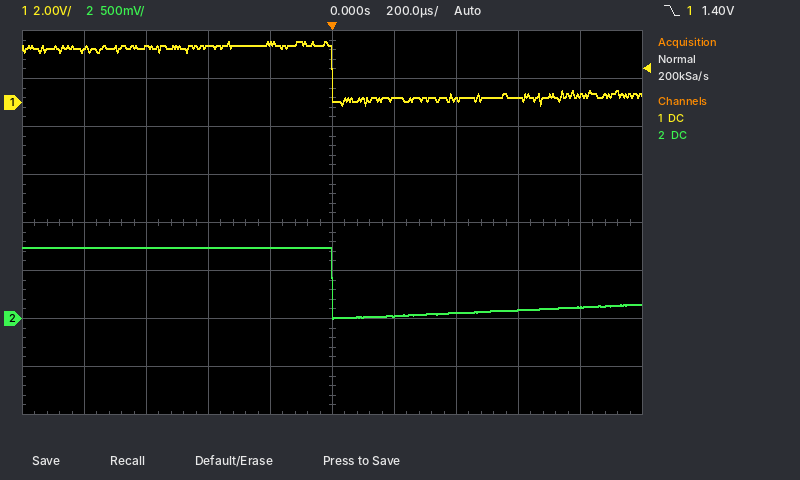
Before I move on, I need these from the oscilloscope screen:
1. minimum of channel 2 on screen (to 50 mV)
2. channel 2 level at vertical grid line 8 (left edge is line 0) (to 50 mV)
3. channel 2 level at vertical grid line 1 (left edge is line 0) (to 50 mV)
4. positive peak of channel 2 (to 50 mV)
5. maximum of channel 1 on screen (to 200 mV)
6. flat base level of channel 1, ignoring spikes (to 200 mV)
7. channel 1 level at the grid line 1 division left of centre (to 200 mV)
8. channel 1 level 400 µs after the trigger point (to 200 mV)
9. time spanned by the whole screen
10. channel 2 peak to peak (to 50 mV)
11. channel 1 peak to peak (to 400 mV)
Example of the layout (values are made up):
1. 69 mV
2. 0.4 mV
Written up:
1. 0 mV
2. 100 mV
3. 750 mV
4. 750 mV
5. 2.6 V
6. 200 mV
7. 2.4 V
8. 200 mV
9. 2 ms
10. 750 mV
11. 2.8 V
